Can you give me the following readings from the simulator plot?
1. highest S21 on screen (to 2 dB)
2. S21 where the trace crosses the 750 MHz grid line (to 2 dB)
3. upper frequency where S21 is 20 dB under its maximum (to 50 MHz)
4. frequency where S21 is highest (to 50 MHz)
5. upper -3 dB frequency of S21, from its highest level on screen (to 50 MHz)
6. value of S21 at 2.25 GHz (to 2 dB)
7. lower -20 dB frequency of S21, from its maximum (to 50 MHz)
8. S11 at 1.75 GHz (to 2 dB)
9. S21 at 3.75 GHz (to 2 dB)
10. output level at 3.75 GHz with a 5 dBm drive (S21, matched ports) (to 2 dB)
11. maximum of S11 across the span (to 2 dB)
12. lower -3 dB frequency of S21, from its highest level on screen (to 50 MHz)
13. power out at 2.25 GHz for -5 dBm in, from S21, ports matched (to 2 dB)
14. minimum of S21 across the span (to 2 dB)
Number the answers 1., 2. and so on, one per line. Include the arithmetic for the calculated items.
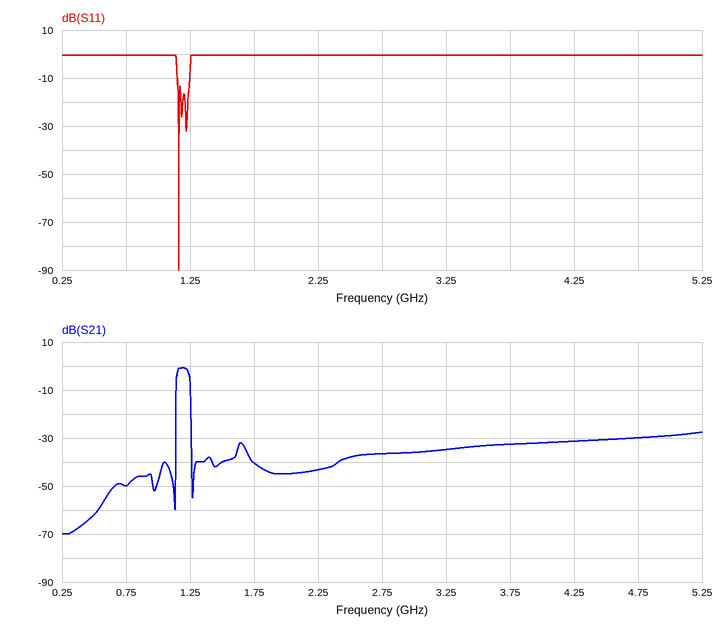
1. 0 dB
2. -50 dB
3. 1.25 GHz
4. 1.20 GHz
5. 1.25 GHz
6. -44 dB
7. 1.15 GHz
8. 0 dB
9. -32 dB
10. 5 dBm + (-32 dB) = -28 dBm
11. 0 dB
12. 1.15 GHz
13. -5 dBm + (-44 dB) = -48 dBm
14. -70 dB
